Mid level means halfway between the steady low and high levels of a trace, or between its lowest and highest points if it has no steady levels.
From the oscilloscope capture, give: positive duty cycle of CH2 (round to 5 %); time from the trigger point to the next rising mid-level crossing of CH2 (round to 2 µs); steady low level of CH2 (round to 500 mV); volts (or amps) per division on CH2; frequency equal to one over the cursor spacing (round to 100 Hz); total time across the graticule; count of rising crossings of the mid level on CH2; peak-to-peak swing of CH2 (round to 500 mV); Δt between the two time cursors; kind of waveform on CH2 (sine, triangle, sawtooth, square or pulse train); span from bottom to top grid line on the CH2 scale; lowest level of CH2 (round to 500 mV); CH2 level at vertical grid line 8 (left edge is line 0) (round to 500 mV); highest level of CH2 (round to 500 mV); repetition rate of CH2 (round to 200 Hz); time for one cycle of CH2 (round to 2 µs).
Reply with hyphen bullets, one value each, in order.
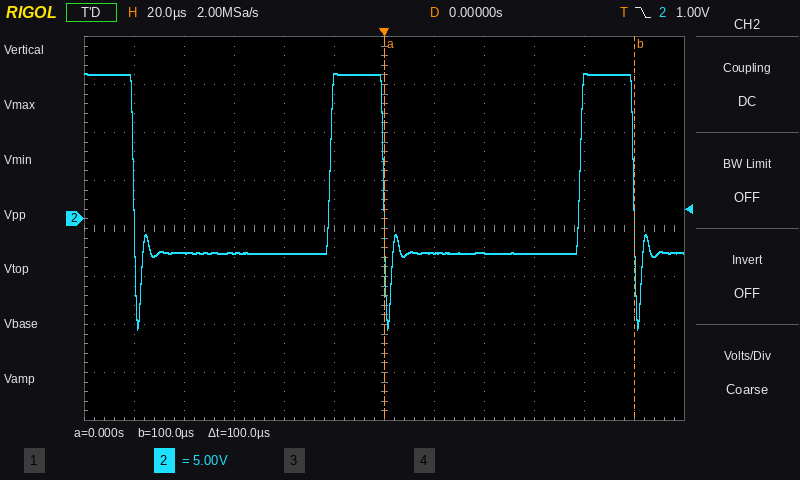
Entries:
- 20 %
- 78 µs
- -3.5 V
- 5 V
- 10.0 kHz
- 240 µs
- 2
- 26.5 V
- 100 µs
- pulse train
- 40 V
- -11.5 V
- -3.5 V
- 15.0 V
- 10.0 kHz
- 100 µs
